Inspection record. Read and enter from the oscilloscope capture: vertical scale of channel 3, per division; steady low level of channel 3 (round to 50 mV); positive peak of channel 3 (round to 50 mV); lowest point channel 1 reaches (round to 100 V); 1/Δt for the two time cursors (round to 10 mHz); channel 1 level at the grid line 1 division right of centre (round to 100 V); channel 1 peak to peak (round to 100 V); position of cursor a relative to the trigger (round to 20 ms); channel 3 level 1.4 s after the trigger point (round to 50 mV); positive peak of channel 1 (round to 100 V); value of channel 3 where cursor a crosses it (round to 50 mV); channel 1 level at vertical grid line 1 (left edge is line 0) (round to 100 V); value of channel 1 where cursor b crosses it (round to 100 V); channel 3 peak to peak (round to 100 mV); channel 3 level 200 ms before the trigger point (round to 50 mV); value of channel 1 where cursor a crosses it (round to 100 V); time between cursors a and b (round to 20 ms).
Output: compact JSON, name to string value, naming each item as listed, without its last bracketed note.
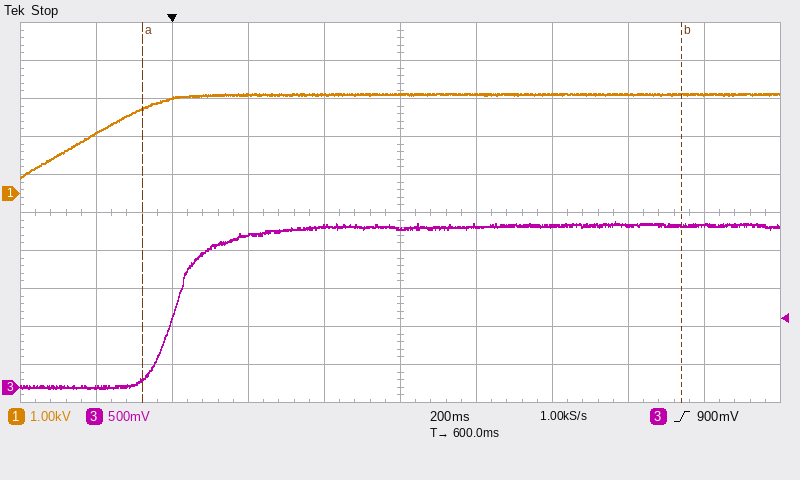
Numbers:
{"vertical scale of channel 3, per division": "500 mV", "steady low level of channel 3": "0 mV", "positive peak of channel 3": "2.20 V", "lowest point channel 1 reaches": "400 V", "1/Δt for the two time cursors": "700 mHz", "channel 1 level at the grid line 1 division right of centre": "2.6 kV", "channel 1 peak to peak": "2.2 kV", "position of cursor a relative to the trigger": "-80 ms", "channel 3 level 1.4 s after the trigger point": "2.15 V", "positive peak of channel 1": "2.6 kV", "value of channel 3 where cursor a crosses it": "100 mV", "channel 1 level at vertical grid line 1 (left edge is line 0)": "1.6 kV", "value of channel 1 where cursor b crosses it": "2.6 kV", "channel 3 peak to peak": "2.20 V", "channel 3 level 200 ms before the trigger point": "0 mV", "value of channel 1 where cursor a crosses it": "2.2 kV", "time between cursors a and b": "1.42 s"}
